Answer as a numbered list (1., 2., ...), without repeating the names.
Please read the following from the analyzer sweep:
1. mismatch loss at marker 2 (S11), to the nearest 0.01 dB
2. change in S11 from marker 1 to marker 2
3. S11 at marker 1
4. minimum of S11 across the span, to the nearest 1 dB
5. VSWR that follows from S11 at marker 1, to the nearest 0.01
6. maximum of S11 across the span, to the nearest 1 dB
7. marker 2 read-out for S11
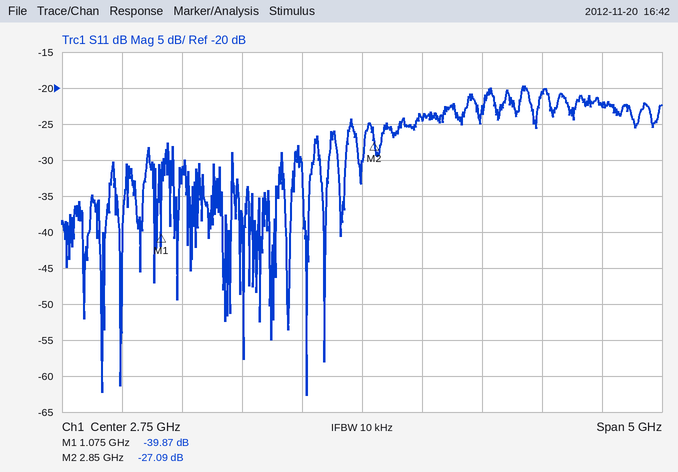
1. 0.01 dB
2. 12.78 dB
3. -39.87 dB
4. -63 dB
5. 1.02
6. -20 dB
7. -27.09 dB
